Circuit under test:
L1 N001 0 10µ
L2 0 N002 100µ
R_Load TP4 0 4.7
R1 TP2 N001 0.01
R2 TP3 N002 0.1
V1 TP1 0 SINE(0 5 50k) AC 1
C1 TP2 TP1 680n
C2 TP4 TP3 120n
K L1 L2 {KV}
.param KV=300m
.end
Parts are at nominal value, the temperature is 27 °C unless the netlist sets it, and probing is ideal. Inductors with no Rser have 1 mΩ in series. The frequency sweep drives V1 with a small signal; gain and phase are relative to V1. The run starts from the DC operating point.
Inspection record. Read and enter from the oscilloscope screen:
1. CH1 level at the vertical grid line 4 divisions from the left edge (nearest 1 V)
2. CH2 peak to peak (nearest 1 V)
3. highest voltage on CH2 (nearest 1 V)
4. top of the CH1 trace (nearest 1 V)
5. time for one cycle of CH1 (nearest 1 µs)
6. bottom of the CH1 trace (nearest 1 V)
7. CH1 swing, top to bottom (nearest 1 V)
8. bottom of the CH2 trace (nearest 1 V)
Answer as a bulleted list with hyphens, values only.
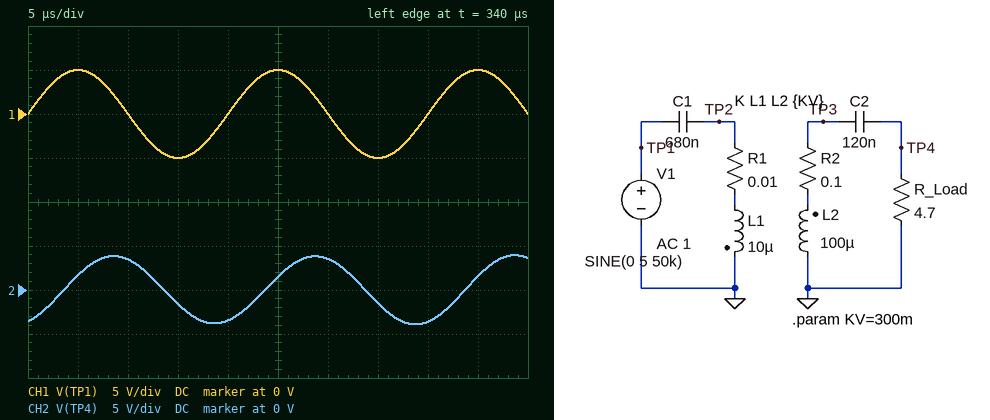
- 0 V
- 8 V
- 4 V
- 5 V
- 20 µs
- -5 V
- 10 V
- -4 V
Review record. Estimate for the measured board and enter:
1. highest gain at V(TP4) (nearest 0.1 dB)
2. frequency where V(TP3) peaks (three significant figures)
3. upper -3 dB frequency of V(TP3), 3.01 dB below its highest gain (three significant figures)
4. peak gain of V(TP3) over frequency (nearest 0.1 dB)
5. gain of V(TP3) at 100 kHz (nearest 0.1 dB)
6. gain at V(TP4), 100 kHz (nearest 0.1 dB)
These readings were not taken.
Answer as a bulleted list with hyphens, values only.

- 14.3 dB
- 66.7 kHz
- 68.0 kHz
- 27.0 dB
- -5.7 dB
- -15.2 dB
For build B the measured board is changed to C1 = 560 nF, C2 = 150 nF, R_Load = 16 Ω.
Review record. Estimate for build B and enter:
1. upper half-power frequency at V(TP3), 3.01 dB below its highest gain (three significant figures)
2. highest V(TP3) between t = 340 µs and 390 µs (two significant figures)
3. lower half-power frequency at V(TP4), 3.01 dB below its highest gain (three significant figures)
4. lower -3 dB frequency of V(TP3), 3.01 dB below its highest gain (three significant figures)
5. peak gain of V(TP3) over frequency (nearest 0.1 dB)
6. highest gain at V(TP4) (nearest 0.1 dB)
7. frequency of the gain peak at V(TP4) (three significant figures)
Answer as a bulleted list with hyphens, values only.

- 73.4 kHz
- 7.4 V
- 68.8 kHz
- 68.7 kHz
- 20.3 dB
- 17.6 dB
- 71.1 kHz
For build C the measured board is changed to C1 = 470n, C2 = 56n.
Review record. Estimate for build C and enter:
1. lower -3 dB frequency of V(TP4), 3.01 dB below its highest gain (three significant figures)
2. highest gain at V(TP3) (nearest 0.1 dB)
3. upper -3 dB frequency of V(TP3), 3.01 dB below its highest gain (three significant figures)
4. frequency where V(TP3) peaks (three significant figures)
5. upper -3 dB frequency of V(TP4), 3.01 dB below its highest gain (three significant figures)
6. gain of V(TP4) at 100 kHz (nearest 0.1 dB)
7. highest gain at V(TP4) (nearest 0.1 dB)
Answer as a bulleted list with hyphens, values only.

- 81.8 kHz
- 28.6 dB
- 86.2 kHz
- 84.1 kHz
- 86.3 kHz
- -7.4 dB
- 11.4 dB
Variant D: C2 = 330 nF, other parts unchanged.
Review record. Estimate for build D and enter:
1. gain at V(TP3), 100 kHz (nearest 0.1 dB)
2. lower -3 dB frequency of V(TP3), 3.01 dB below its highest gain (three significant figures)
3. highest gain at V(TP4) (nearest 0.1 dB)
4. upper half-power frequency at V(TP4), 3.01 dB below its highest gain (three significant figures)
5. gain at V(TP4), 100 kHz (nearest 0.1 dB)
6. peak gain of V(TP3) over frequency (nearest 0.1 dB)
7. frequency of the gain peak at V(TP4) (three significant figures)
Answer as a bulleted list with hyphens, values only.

- -13.7 dB
- 64.0 kHz
- 17.2 dB
- 65.3 kHz
- -16.8 dB
- 22.7 dB
- 64.6 kHz
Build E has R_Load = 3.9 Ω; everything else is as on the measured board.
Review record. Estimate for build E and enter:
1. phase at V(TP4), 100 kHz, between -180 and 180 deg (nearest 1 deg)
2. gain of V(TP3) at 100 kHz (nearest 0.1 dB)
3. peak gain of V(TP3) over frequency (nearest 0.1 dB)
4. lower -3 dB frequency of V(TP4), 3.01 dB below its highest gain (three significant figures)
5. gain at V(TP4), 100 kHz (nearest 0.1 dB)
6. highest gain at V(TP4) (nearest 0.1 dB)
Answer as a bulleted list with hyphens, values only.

- 96 deg
- -5.8 dB
- 28.4 dB
- 65.7 kHz
- -16.8 dB
- 14.1 dB
